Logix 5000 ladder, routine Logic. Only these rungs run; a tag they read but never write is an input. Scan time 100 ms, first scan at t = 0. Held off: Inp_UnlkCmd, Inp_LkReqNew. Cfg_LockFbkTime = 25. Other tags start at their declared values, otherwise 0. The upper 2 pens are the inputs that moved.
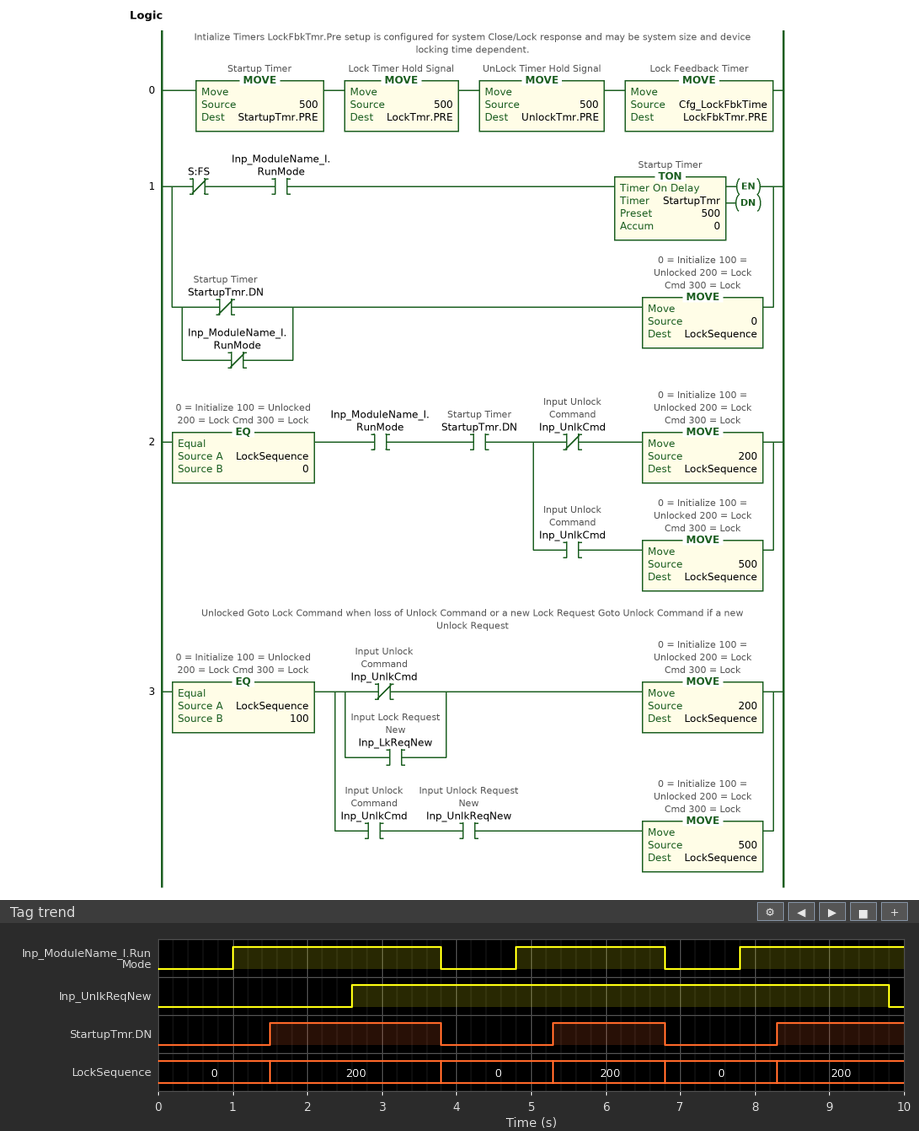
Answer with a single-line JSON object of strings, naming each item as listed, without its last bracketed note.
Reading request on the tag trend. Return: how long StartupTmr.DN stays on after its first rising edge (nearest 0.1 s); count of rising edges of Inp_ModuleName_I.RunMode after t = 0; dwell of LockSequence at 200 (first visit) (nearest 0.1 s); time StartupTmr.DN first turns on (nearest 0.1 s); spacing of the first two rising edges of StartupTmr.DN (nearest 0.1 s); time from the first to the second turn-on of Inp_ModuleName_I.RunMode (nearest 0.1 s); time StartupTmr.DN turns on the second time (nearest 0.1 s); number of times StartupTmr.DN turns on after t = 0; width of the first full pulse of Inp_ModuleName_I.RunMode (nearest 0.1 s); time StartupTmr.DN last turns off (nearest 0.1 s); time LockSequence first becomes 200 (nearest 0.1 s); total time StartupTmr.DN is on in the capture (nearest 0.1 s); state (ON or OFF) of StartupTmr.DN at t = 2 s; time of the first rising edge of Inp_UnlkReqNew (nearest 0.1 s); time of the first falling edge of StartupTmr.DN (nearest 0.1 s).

{"how long StartupTmr.DN stays on after its first rising edge": "2.3 s", "count of rising edges of Inp_ModuleName_I.RunMode after t = 0": "3", "dwell of LockSequence at 200 (first visit)": "2.3 s", "time StartupTmr.DN first turns on": "1.5 s", "spacing of the first two rising edges of StartupTmr.DN": "3.8 s", "time from the first to the second turn-on of Inp_ModuleName_I.RunMode": "3.8 s", "time StartupTmr.DN turns on the second time": "5.3 s", "number of times StartupTmr.DN turns on after t = 0": "3", "width of the first full pulse of Inp_ModuleName_I.RunMode": "2.8 s", "time StartupTmr.DN last turns off": "6.8 s", "time LockSequence first becomes 200": "1.5 s", "total time StartupTmr.DN is on in the capture": "5.5 s", "state (ON or OFF) of StartupTmr.DN at t = 2 s": "ON", "time of the first rising edge of Inp_UnlkReqNew": "2.6 s", "time of the first falling edge of StartupTmr.DN": "3.8 s"}
